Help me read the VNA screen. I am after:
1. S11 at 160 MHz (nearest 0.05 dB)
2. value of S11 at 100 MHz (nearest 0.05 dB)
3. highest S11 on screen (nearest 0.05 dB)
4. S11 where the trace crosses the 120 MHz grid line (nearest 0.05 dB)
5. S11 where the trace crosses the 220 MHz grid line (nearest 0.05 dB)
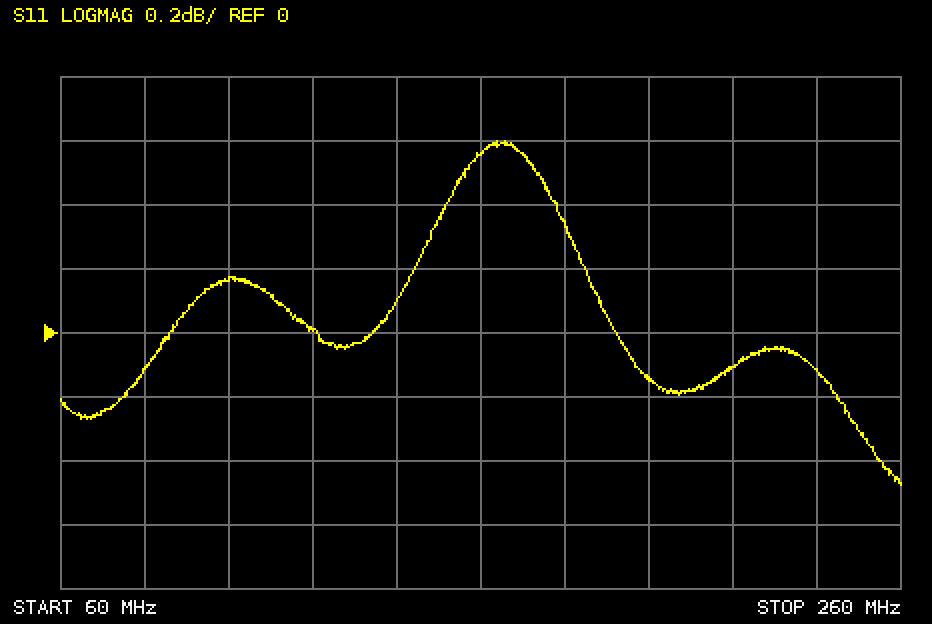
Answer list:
0.55 dB
0.15 dB
0.60 dB
0.00 dB
-0.10 dB
